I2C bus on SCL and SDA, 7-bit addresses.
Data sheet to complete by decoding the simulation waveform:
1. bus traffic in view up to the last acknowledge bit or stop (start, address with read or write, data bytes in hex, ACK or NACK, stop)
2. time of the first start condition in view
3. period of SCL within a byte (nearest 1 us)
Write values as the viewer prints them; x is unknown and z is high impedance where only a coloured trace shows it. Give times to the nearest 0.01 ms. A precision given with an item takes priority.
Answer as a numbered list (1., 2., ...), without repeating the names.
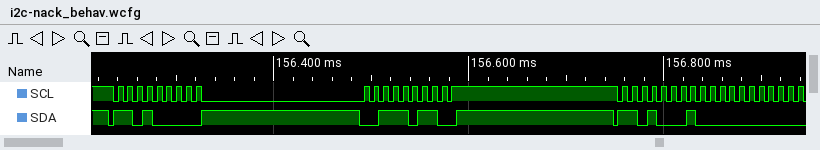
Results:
1. start, address 68 write ACK, 3B ACK, stop, start, address 68 read ACK, 00 ACK
2. 156.23 ms
3. 10 us
